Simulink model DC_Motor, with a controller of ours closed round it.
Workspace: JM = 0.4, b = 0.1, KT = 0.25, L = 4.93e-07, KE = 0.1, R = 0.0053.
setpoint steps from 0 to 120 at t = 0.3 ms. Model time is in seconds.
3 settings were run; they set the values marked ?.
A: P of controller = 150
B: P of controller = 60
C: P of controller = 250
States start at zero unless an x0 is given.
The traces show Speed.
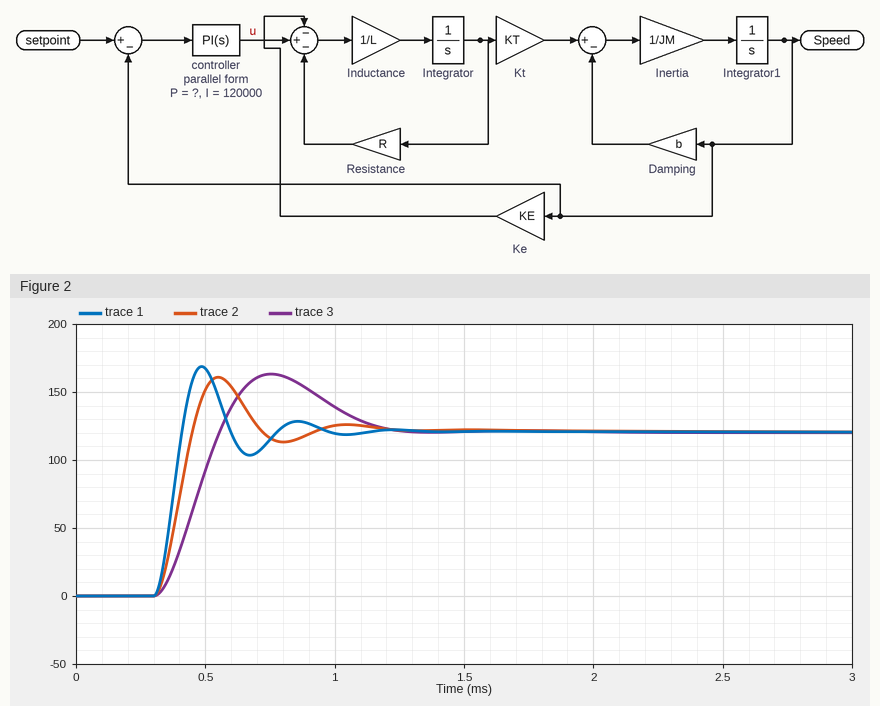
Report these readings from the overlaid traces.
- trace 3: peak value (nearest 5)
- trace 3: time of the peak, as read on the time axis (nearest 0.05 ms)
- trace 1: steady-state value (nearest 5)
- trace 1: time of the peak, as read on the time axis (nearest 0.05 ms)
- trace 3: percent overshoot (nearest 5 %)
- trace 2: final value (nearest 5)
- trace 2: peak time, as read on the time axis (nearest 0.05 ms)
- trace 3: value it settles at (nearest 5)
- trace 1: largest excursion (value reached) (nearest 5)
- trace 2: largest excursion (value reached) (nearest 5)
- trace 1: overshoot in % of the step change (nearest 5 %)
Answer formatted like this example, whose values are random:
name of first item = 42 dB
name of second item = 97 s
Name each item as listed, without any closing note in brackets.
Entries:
trace 3: peak value = 165
trace 3: time of the peak, as read on the time axis = 0.75 ms
trace 1: steady-state value = 120
trace 1: time of the peak, as read on the time axis = 0.50 ms
trace 3: percent overshoot = 35 %
trace 2: final value = 120
trace 2: peak time, as read on the time axis = 0.55 ms
trace 3: value it settles at = 120
trace 1: largest excursion (value reached) = 170
trace 2: largest excursion (value reached) = 160
trace 1: overshoot in % of the step change = 40 %
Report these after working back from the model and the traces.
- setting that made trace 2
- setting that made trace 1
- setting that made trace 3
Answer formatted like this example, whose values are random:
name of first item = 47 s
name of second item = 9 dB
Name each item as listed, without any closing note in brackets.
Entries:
setting that made trace 2 = A
setting that made trace 1 = C
setting that made trace 3 = B
